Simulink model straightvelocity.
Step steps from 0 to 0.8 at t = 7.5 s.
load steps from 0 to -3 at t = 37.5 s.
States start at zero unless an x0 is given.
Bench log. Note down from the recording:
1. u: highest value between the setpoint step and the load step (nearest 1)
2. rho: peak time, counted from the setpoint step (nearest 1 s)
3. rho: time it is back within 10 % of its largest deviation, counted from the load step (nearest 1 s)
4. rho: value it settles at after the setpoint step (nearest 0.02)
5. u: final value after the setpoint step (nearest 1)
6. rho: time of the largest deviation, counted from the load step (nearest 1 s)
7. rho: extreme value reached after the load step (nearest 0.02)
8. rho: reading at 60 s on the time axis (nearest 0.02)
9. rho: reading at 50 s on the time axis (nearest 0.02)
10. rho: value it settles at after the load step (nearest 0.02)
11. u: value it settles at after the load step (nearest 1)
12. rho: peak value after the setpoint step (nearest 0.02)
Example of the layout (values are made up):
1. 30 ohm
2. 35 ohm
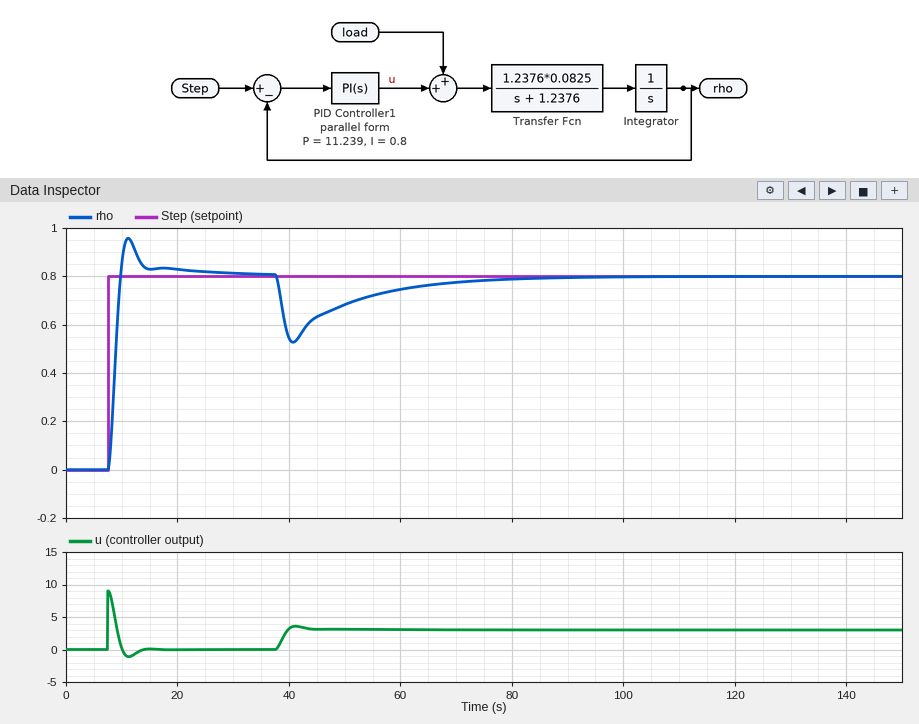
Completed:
1. 9
2. 4 s
3. 31 s
4. 0.80
5. 0
6. 3 s
7. 0.52
8. 0.74
9. 0.68
10. 0.80
11. 3
12. 0.96
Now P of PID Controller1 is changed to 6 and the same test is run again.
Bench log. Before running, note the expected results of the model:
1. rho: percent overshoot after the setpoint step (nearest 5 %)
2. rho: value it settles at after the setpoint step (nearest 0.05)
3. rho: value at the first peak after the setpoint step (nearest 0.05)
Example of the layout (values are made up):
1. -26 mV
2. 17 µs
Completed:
1. 25 %
2. 0.80
3. 1.00
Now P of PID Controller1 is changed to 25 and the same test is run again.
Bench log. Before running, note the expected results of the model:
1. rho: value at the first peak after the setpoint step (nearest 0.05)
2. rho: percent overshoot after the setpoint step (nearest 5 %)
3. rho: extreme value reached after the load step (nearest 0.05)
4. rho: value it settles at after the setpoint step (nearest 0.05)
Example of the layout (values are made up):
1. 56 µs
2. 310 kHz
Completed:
1. 1.05
2. 30 %
3. 0.65
4. 0.80
